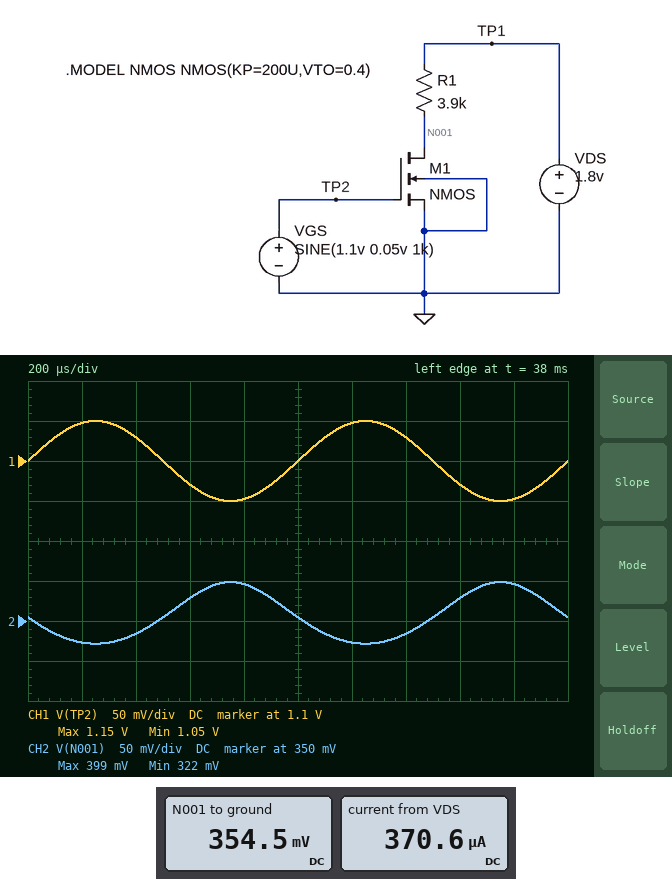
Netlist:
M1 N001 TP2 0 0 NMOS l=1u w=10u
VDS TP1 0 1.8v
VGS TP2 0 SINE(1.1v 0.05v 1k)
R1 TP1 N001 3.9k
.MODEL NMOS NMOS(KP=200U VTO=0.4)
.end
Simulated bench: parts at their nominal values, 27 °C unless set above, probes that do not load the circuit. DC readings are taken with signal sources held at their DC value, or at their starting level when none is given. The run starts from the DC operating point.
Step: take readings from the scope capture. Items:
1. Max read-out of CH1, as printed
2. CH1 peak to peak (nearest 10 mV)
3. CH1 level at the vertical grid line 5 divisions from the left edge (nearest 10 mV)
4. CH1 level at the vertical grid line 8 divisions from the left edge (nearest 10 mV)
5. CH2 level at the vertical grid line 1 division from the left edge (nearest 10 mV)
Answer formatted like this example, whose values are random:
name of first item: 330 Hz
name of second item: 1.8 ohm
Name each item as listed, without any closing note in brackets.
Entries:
Max read-out of CH1, as printed: 1.15 V
CH1 peak to peak: 100 mV
CH1 level at the vertical grid line 5 divisions from the left edge: 1.10 V
CH1 level at the vertical grid line 8 divisions from the left edge: 1.07 V
CH2 level at the vertical grid line 1 division from the left edge: 320 mV
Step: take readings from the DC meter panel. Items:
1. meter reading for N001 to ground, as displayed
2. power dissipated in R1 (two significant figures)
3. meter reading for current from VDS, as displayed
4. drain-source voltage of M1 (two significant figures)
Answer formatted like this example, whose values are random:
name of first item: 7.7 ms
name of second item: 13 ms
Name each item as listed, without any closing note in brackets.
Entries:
meter reading for N001 to ground, as displayed: 354.5 mV
power dissipated in R1: 540 µW
meter reading for current from VDS, as displayed: 370.6 µA
drain-source voltage of M1: 350 mV
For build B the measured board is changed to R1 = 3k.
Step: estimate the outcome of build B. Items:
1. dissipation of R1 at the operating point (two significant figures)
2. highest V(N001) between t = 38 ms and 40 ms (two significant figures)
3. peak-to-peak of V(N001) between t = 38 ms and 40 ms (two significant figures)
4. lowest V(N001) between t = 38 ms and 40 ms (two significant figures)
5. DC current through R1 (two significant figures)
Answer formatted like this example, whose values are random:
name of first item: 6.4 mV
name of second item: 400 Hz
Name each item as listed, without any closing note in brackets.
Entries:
dissipation of R1 at the operating point: 580 µW
highest V(N001) between t = 38 ms and 40 ms: 560 mV
peak-to-peak of V(N001) between t = 38 ms and 40 ms: 130 mV
lowest V(N001) between t = 38 ms and 40 ms: 430 mV
DC current through R1: 440 µA
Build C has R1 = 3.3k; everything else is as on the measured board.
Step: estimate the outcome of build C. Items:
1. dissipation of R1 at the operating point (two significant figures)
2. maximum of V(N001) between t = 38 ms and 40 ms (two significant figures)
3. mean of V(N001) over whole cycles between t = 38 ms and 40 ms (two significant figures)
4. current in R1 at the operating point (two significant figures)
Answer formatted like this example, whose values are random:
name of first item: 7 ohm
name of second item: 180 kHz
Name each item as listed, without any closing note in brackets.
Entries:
dissipation of R1 at the operating point: 570 µW
maximum of V(N001) between t = 38 ms and 40 ms: 490 mV
mean of V(N001) over whole cycles between t = 38 ms and 40 ms: 430 mV
current in R1 at the operating point: 420 µA
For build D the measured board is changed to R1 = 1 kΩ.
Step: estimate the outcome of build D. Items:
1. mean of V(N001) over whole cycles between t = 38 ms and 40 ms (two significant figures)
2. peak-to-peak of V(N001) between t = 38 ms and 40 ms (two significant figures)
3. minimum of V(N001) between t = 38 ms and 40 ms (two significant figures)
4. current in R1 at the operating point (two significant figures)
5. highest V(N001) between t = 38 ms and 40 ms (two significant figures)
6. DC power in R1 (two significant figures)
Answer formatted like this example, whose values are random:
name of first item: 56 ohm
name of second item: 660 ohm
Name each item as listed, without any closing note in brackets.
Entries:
mean of V(N001) over whole cycles between t = 38 ms and 40 ms: 1.3 V
peak-to-peak of V(N001) between t = 38 ms and 40 ms: 140 mV
minimum of V(N001) between t = 38 ms and 40 ms: 1.2 V
current in R1 at the operating point: 490 µA
highest V(N001) between t = 38 ms and 40 ms: 1.4 V
DC power in R1: 240 µW
